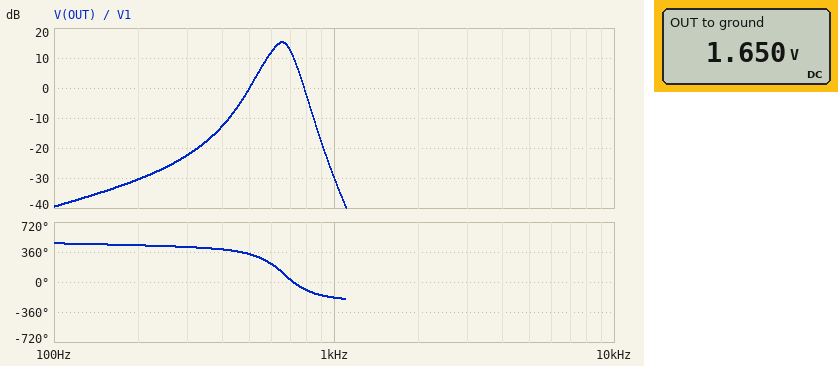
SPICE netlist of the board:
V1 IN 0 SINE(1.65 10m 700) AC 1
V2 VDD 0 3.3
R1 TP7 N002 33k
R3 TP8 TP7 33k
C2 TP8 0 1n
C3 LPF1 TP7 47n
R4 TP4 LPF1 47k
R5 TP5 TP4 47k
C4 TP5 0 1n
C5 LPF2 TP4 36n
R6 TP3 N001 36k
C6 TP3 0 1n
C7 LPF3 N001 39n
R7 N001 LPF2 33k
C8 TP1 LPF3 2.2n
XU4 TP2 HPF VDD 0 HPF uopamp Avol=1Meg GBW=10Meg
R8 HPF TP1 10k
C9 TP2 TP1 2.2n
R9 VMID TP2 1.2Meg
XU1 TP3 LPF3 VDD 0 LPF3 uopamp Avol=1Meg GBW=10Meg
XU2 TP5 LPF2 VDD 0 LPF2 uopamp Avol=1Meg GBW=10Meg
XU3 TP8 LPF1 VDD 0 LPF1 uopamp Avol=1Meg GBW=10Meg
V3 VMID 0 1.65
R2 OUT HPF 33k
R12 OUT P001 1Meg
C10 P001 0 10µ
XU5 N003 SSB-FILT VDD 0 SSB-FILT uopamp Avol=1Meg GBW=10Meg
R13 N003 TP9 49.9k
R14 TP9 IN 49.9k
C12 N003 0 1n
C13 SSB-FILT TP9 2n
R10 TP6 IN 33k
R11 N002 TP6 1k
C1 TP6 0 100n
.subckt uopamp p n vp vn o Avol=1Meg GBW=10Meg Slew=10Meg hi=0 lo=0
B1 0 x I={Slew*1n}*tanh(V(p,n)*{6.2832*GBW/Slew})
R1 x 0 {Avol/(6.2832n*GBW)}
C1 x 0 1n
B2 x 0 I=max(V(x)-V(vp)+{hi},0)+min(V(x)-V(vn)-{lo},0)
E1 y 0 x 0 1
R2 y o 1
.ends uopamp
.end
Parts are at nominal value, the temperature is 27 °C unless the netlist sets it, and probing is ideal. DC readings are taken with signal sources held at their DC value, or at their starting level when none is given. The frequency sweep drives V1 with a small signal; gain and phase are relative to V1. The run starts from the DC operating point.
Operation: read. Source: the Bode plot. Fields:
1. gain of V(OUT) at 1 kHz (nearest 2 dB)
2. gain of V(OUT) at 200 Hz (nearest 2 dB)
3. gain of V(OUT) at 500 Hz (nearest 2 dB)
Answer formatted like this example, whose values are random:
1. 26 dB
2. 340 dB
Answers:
1. -30 dB
2. -30 dB
3. 0 dB
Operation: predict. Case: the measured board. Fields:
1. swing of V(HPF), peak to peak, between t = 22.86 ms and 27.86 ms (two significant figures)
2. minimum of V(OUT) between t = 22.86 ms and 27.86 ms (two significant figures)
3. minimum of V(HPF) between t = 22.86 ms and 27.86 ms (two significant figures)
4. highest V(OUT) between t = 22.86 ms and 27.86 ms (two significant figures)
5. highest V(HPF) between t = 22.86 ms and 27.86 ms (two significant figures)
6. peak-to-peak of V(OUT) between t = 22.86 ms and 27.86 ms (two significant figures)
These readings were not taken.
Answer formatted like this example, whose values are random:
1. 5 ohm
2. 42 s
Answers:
1. 85 mV
2. 1.6 V
3. 1.6 V
4. 1.7 V
5. 1.7 V
6. 82 mV
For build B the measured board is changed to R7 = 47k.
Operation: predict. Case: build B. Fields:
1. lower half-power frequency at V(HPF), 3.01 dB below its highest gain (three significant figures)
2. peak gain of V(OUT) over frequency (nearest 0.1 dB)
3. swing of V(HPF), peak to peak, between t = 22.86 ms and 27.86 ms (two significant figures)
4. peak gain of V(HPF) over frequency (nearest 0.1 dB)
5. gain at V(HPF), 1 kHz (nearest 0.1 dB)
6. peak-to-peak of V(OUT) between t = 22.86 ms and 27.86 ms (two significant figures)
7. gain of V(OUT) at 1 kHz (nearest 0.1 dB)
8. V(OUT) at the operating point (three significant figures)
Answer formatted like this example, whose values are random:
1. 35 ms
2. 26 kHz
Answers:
1. 577 Hz
2. 15.9 dB
3. 59 mV
4. 16.2 dB
5. -34.6 dB
6. 57 mV
7. -34.9 dB
8. 1.65 V
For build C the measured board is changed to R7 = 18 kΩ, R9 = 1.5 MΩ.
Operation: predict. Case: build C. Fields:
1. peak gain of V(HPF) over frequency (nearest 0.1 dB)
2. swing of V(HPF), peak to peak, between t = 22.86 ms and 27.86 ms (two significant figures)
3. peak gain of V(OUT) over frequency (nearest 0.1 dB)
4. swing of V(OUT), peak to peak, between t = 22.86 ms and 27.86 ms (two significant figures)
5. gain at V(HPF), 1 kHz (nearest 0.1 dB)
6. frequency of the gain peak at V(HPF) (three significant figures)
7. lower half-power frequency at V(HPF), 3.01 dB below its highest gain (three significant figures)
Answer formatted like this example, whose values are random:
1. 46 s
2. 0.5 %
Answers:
1. 13.8 dB
2. 31 mV
3. 13.5 dB
4. 30 mV
5. -21.8 dB
6. 591 Hz
7. 552 Hz
